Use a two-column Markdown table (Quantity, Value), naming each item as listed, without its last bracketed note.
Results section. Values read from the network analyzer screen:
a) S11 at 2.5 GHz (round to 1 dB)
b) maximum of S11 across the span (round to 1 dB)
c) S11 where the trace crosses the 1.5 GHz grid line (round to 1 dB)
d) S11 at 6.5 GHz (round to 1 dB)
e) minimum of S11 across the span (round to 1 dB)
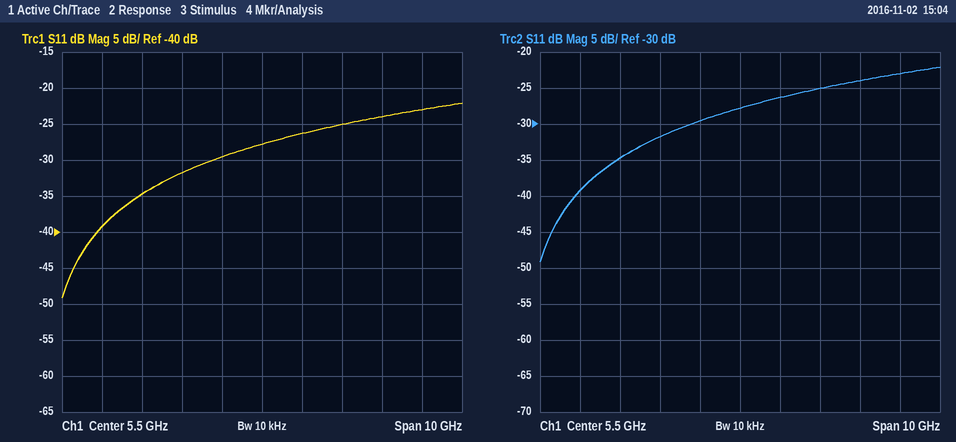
| Quantity | Value |
|---|---|
| S11 at 2.5 GHz | -35 dB |
| maximum of S11 across the span | -22 dB |
| S11 where the trace crosses the 1.5 GHz grid line | -39 dB |
| S11 at 6.5 GHz | -26 dB |
| minimum of S11 across the span | -49 dB |
